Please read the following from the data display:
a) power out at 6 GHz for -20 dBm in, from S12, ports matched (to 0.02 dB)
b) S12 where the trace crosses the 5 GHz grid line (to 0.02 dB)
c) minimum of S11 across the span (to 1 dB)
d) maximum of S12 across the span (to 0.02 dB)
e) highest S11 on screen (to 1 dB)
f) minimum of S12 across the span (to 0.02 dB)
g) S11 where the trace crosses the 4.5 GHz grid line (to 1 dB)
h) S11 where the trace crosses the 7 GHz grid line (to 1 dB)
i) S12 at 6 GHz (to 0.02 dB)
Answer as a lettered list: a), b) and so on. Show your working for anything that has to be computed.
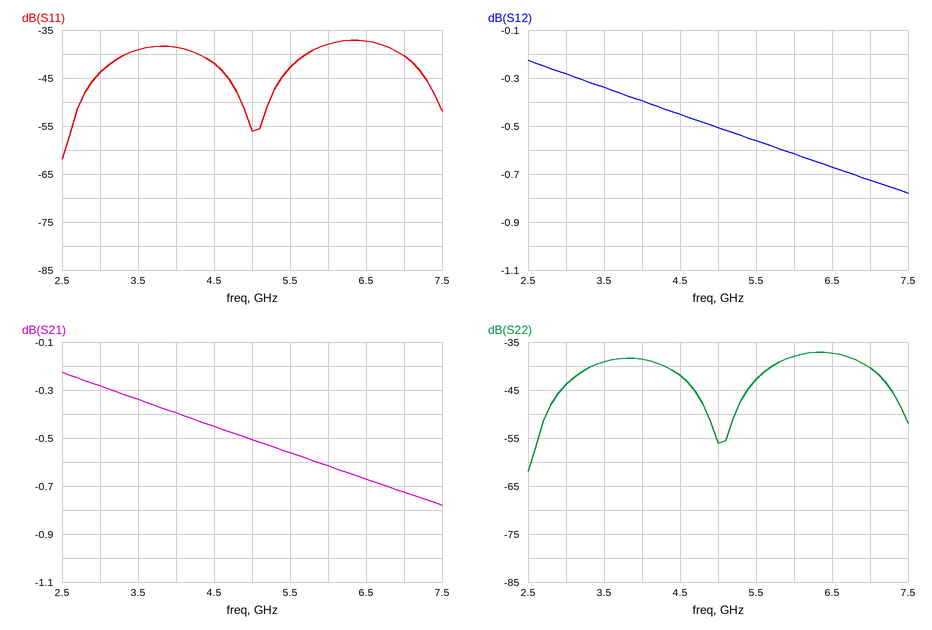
a) -20 dBm + (-0.62 dB) = -20.62 dBm
b) -0.50 dB
c) -62 dB
d) -0.22 dB
e) -37 dB
f) -0.78 dB
g) -42 dB
h) -40 dB
i) -0.62 dB
